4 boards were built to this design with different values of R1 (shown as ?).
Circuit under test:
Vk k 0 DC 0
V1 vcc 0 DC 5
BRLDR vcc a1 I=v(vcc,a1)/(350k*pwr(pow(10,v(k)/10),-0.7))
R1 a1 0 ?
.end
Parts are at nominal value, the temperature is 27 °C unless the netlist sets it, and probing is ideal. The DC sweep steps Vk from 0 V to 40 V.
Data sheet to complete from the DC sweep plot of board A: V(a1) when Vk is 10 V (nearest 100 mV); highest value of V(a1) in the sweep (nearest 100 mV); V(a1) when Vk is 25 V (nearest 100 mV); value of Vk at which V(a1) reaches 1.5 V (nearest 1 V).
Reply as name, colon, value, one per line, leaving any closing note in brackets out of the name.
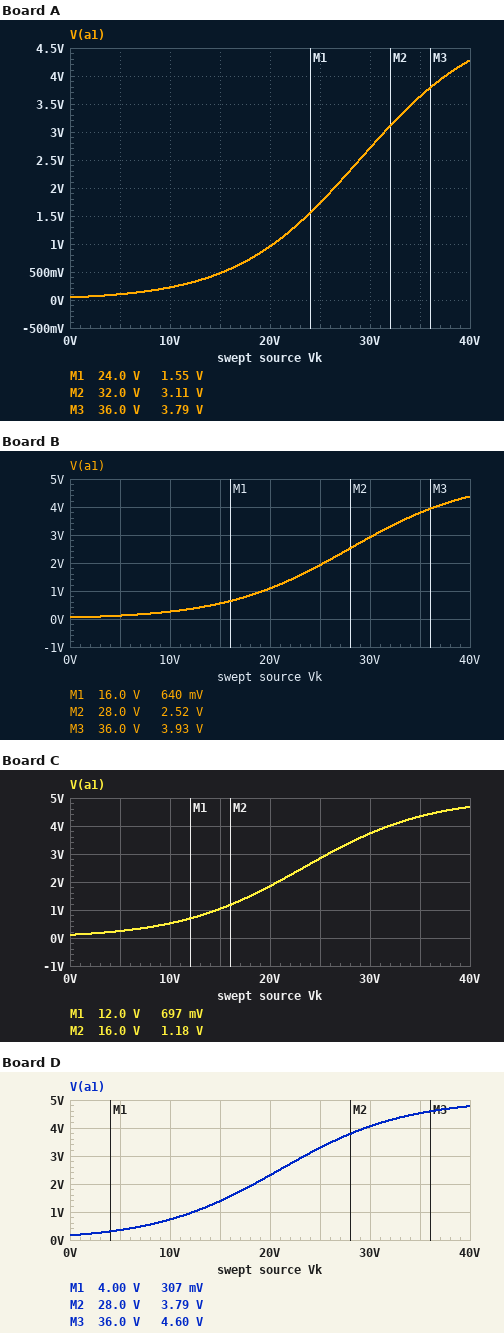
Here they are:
V(a1) when Vk is 10 V: 200 mV
highest value of V(a1) in the sweep: 4.3 V
V(a1) when Vk is 25 V: 1.7 V
value of Vk at which V(a1) reaches 1.5 V: 24 V
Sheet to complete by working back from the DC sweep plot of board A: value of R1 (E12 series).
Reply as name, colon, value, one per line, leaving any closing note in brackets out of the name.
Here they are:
value of R1: 3.3 kΩ
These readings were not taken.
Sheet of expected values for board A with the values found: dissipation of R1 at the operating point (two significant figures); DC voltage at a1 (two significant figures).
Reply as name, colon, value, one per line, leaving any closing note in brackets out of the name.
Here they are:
dissipation of R1 at the operating point: 660 nW
DC voltage at a1: 47 mV
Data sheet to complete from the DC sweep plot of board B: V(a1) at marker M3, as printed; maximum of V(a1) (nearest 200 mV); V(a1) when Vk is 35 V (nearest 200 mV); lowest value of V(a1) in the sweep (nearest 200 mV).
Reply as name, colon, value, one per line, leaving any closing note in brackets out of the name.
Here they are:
V(a1) at marker M3, as printed: 3.93 V
maximum of V(a1): 4.4 V
V(a1) when Vk is 35 V: 3.8 V
lowest value of V(a1) in the sweep: 0 V
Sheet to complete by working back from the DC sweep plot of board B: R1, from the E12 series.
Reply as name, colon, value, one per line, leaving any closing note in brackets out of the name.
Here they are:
R1, from the E12 series: 3.9 kΩ
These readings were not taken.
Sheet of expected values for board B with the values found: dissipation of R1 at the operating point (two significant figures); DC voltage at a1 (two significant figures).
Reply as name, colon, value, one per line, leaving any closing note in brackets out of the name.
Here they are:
dissipation of R1 at the operating point: 780 nW
DC voltage at a1: 55 mV
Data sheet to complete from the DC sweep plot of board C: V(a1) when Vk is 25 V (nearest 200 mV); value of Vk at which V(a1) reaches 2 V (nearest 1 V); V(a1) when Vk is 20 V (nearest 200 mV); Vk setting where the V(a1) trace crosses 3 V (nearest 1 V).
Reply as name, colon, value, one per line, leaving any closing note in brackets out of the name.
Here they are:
V(a1) when Vk is 25 V: 2.8 V
value of Vk at which V(a1) reaches 2 V: 21 V
V(a1) when Vk is 20 V: 1.8 V
Vk setting where the V(a1) trace crosses 3 V: 26 V
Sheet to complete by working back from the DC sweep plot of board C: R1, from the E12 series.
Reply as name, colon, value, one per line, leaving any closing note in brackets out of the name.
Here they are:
R1, from the E12 series: 8.2 kΩ
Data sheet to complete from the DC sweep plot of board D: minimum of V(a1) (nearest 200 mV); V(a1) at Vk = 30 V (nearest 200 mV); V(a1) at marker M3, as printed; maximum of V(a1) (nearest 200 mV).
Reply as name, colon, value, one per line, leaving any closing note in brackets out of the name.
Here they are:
minimum of V(a1): 200 mV
V(a1) at Vk = 30 V: 4.0 V
V(a1) at marker M3, as printed: 4.60 V
maximum of V(a1): 4.8 V
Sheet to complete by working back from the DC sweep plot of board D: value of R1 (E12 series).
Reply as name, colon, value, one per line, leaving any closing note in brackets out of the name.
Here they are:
value of R1: 12 kΩ
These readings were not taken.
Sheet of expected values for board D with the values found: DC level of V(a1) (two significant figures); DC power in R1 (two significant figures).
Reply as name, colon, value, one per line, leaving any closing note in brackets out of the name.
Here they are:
DC level of V(a1): 170 mV
DC power in R1: 2.3 µW
